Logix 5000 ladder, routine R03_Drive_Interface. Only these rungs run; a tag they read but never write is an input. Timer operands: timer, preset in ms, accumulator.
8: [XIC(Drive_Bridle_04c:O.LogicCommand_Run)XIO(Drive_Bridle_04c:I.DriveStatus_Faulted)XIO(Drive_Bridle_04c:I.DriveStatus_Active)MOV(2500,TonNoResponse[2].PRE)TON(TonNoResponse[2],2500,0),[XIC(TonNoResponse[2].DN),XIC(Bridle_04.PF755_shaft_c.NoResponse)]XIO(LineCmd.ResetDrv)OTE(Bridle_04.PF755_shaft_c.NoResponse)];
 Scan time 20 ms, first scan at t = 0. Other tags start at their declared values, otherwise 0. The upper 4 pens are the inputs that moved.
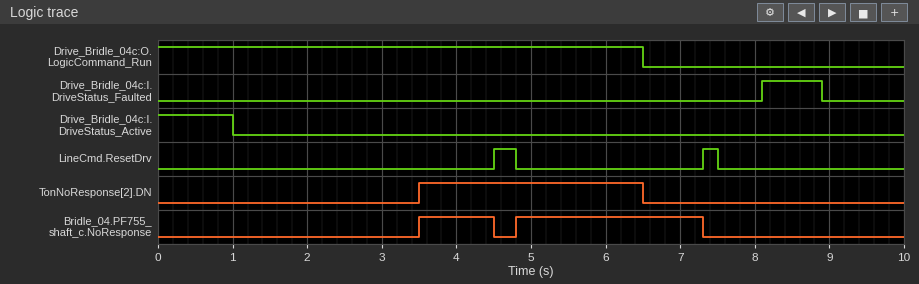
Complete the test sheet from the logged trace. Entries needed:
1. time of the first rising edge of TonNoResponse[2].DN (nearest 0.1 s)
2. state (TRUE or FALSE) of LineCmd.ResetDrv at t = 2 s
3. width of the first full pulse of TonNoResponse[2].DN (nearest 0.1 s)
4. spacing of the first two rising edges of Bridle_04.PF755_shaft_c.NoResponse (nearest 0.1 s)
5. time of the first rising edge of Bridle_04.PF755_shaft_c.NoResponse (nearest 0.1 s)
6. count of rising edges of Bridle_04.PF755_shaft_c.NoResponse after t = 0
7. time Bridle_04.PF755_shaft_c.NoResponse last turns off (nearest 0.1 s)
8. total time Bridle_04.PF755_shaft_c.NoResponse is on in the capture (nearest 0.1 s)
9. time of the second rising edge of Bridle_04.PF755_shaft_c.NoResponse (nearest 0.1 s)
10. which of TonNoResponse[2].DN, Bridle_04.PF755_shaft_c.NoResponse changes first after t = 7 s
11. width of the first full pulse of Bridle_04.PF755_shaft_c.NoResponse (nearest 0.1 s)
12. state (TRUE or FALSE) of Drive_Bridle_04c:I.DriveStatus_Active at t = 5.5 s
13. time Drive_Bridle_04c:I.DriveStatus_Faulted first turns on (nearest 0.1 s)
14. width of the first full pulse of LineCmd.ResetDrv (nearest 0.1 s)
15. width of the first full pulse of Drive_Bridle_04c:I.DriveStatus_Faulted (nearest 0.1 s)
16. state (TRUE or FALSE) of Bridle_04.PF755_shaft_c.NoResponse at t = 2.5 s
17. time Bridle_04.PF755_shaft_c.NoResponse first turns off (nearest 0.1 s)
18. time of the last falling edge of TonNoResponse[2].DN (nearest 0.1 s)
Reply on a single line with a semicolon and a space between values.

3.5 s; FALSE; 3.0 s; 1.3 s; 3.5 s; 2; 7.3 s; 3.5 s; 4.8 s; Bridle_04.PF755_shaft_c.NoResponse; 1.0 s; FALSE; 8.1 s; 0.3 s; 0.8 s; FALSE; 4.5 s; 6.5 s
